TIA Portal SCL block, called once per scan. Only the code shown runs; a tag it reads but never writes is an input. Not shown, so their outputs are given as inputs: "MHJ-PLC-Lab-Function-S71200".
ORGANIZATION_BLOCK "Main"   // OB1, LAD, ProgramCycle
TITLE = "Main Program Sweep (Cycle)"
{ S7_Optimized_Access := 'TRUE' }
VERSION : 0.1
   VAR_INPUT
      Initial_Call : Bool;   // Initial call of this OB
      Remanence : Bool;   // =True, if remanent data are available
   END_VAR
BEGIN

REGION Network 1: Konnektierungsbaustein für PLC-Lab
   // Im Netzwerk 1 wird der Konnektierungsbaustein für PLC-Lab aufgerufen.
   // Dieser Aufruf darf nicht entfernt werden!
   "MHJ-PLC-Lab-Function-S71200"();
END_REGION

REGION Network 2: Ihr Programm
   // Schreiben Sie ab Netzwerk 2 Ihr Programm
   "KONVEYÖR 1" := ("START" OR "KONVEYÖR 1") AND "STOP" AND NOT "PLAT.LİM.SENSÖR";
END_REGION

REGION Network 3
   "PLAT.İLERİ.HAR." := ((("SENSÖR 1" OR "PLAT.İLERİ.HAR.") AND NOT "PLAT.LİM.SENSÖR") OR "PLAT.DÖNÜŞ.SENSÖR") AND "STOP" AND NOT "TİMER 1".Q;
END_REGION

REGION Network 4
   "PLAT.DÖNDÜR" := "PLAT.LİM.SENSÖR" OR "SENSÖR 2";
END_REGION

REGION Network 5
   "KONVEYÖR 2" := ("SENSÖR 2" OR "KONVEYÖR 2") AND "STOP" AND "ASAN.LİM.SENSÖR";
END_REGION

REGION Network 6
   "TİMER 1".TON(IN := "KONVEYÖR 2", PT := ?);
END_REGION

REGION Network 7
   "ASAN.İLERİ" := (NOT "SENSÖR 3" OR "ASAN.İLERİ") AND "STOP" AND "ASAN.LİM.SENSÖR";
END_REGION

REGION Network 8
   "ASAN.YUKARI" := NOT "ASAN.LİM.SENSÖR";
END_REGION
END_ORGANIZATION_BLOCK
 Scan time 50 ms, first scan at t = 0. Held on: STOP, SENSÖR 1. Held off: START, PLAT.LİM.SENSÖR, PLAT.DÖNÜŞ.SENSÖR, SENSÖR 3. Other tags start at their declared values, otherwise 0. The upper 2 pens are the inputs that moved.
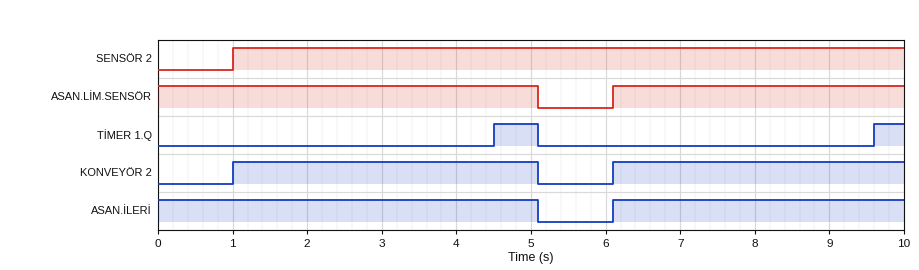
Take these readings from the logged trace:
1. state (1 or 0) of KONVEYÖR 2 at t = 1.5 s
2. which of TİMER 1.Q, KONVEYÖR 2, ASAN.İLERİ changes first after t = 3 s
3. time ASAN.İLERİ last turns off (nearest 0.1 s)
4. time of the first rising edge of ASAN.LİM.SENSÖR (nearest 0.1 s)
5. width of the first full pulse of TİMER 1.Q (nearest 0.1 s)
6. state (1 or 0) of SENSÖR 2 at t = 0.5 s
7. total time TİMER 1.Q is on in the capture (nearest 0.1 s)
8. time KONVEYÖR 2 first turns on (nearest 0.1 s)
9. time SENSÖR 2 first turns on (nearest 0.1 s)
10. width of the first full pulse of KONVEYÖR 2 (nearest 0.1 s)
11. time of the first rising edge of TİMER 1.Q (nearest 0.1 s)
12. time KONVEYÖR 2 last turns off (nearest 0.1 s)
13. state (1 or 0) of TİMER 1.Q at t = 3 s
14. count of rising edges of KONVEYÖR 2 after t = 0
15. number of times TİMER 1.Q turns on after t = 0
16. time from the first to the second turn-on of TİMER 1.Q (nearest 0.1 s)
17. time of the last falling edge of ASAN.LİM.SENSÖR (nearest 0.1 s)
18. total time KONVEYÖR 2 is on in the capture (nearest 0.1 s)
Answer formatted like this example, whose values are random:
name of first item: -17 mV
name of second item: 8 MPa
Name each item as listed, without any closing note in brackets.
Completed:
state (1 or 0) of KONVEYÖR 2 at t = 1.5 s: 1
which of TİMER 1.Q, KONVEYÖR 2, ASAN.İLERİ changes first after t = 3 s: TİMER 1.Q
time ASAN.İLERİ last turns off: 5.1 s
time of the first rising edge of ASAN.LİM.SENSÖR: 6.1 s
width of the first full pulse of TİMER 1.Q: 0.6 s
state (1 or 0) of SENSÖR 2 at t = 0.5 s: 0
total time TİMER 1.Q is on in the capture: 1.0 s
time KONVEYÖR 2 first turns on: 1.0 s
time SENSÖR 2 first turns on: 1.0 s
width of the first full pulse of KONVEYÖR 2: 4.1 s
time of the first rising edge of TİMER 1.Q: 4.5 s
time KONVEYÖR 2 last turns off: 5.1 s
state (1 or 0) of TİMER 1.Q at t = 3 s: 0
count of rising edges of KONVEYÖR 2 after t = 0: 2
number of times TİMER 1.Q turns on after t = 0: 2
time from the first to the second turn-on of TİMER 1.Q: 5.1 s
time of the last falling edge of ASAN.LİM.SENSÖR: 5.1 s
total time KONVEYÖR 2 is on in the capture: 8.0 s
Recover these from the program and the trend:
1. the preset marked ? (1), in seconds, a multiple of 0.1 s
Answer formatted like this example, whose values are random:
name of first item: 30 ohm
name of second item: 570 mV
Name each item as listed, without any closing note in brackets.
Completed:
the preset marked ? (1), in seconds, a multiple of 0.1 s: 3.5 s
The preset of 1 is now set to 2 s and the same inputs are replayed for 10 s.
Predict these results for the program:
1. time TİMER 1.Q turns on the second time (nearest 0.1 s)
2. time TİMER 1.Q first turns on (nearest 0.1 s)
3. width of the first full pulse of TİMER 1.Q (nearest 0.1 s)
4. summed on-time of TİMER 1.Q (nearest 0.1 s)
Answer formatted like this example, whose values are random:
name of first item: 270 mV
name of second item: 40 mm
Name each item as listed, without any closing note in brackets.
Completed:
time TİMER 1.Q turns on the second time: 8.1 s
time TİMER 1.Q first turns on: 3.0 s
width of the first full pulse of TİMER 1.Q: 2.1 s
summed on-time of TİMER 1.Q: 4.0 s
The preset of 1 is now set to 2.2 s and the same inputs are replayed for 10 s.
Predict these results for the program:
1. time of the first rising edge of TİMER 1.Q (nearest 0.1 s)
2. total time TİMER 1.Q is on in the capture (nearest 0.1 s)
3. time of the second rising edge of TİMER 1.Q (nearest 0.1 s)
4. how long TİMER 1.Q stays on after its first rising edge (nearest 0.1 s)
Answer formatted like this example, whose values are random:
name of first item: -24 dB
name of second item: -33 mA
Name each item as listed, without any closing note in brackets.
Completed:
time of the first rising edge of TİMER 1.Q: 3.2 s
total time TİMER 1.Q is on in the capture: 3.6 s
time of the second rising edge of TİMER 1.Q: 8.3 s
how long TİMER 1.Q stays on after its first rising edge: 1.9 s
